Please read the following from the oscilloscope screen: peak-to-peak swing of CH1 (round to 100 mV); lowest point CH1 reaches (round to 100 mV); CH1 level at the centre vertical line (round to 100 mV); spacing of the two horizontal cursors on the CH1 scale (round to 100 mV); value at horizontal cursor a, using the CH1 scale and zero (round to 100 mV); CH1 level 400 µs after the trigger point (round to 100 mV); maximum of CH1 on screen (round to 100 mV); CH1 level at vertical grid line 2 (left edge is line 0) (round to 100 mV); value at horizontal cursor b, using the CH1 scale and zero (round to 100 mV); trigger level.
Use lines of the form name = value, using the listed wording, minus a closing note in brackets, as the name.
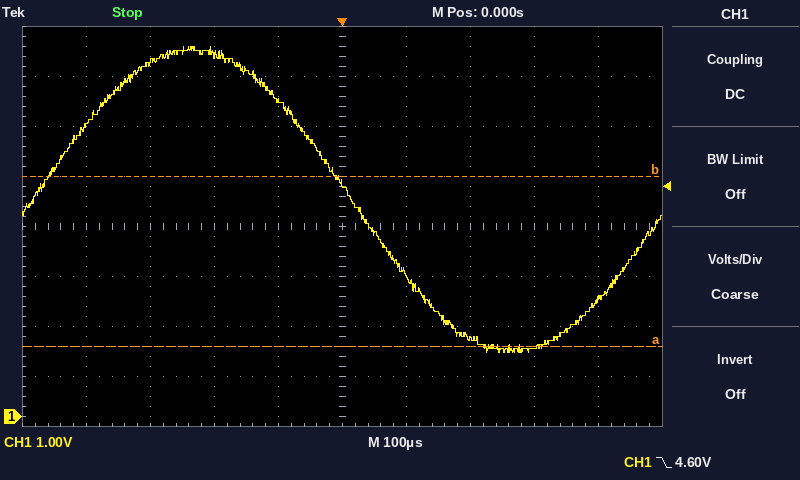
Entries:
peak-to-peak swing of CH1 = 6.1 V
lowest point CH1 reaches = 1.3 V
CH1 level at the centre vertical line = 4.7 V
spacing of the two horizontal cursors on the CH1 scale = 3.4 V
value at horizontal cursor a, using the CH1 scale and zero = 1.4 V
CH1 level 400 µs after the trigger point = 2.3 V
maximum of CH1 on screen = 7.4 V
CH1 level at vertical grid line 2 (left edge is line 0) = 7.1 V
value at horizontal cursor b, using the CH1 scale and zero = 4.8 V
trigger level = 4.60 V
